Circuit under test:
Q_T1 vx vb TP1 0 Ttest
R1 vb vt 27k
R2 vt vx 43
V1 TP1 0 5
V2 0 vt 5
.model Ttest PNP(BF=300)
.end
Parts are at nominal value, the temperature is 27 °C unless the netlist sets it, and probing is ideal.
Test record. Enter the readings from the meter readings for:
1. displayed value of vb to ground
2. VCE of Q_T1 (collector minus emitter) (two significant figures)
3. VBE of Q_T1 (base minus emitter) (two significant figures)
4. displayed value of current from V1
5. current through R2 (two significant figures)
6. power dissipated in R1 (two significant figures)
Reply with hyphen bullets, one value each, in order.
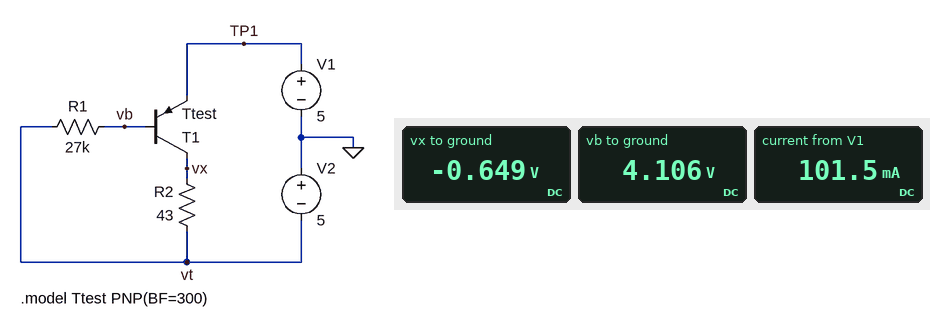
- 4.106 V
- -5.6 V
- -890 mV
- 101.5 mA
- 100 mA
- 3.1 mW
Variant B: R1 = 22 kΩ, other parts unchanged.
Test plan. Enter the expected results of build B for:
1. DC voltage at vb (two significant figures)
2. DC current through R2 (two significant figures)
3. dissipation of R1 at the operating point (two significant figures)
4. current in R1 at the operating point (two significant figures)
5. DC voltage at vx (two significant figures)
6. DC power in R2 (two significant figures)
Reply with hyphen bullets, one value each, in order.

- 4.1 V
- 120 mA
- 3.8 mW
- 410 µA
- 340 mV
- 660 mW
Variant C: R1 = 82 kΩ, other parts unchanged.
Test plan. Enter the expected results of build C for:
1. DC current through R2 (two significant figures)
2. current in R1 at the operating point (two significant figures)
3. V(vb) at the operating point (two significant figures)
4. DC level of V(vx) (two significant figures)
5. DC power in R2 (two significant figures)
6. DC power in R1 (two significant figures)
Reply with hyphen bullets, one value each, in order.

- 33 mA
- 110 µA
- 4.1 V
- -3.6 V
- 48 mW
- 1.0 mW
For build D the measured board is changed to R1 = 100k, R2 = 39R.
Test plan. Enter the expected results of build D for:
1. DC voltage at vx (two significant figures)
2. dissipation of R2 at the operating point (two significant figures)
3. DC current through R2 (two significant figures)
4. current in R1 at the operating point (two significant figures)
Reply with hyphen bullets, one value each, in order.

- -3.9 V
- 29 mW
- 27 mA
- 91 µA
